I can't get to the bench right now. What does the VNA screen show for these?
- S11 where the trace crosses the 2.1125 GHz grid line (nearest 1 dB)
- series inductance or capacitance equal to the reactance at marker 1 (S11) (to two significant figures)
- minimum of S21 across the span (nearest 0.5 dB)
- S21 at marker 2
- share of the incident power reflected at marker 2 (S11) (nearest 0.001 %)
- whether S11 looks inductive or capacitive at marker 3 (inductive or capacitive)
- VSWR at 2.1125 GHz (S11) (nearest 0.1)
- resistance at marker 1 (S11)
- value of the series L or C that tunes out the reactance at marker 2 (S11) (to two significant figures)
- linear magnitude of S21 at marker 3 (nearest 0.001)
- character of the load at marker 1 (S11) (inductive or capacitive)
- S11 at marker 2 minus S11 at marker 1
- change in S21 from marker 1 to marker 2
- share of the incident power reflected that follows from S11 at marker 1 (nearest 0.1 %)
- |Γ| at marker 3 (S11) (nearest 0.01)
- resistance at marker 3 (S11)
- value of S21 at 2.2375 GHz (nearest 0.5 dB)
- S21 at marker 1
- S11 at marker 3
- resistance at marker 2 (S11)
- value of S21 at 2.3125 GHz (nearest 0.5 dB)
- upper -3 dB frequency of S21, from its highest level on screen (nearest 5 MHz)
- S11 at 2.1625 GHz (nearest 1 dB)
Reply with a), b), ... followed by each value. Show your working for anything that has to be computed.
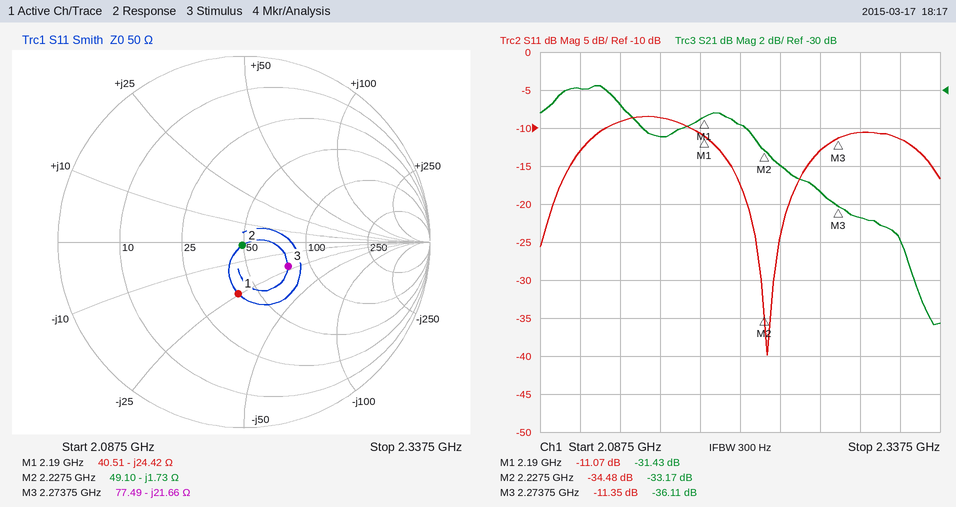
a) -13 dB
b) C = 1/(2π × 2.19 GHz × 24.42 Ω) ≈ 3.0 pF
c) -42.5 dB
d) -33.17 dB
e) 10^(-34.48/10) ≈ 0.036 %
f) capacitive
g) |Γ| = 10^(-13/20) = 0.2239; VSWR = (1 + 0.2239)/(1 − 0.2239) ≈ 1.6
h) 40.51 Ω
i) L = 1.73 Ω/(2π × 2.2275 GHz) ≈ 124 pH, so 120 pH to two significant figures
j) 10^(-36.11/20) ≈ 0.016
k) capacitive
l) -34.48 − (-11.07) = -23.41 dB
m) -33.17 − (-31.43) = -1.74 dB
n) 10^(-11.07/10) ≈ 7.8 %
o) 0.27
p) 77.49 Ω
q) -34.0 dB
r) -31.43 dB
s) -11.35 dB
t) 49.10 Ω
u) -38.0 dB
v) 2.225 GHz
w) -9 dB
